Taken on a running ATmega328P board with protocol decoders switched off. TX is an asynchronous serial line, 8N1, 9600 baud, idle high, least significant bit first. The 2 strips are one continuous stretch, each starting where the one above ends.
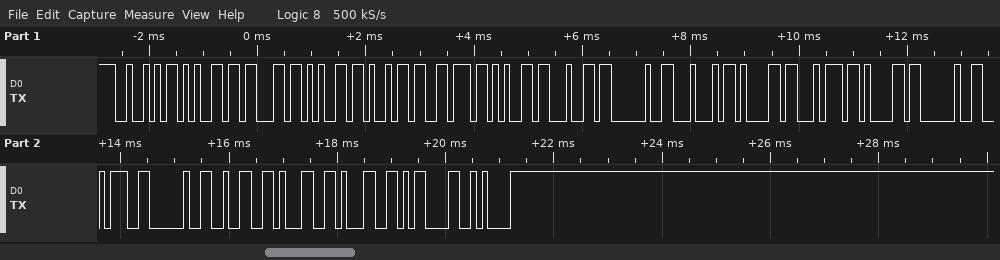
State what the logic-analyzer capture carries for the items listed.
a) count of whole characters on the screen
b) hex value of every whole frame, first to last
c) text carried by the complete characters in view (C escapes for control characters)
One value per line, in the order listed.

21
52 65 63 65 69 76 65 64 20 44 61 74 61 20 3A 20 32 31 31 0D 0A
"Received Data : 211\r\n"
